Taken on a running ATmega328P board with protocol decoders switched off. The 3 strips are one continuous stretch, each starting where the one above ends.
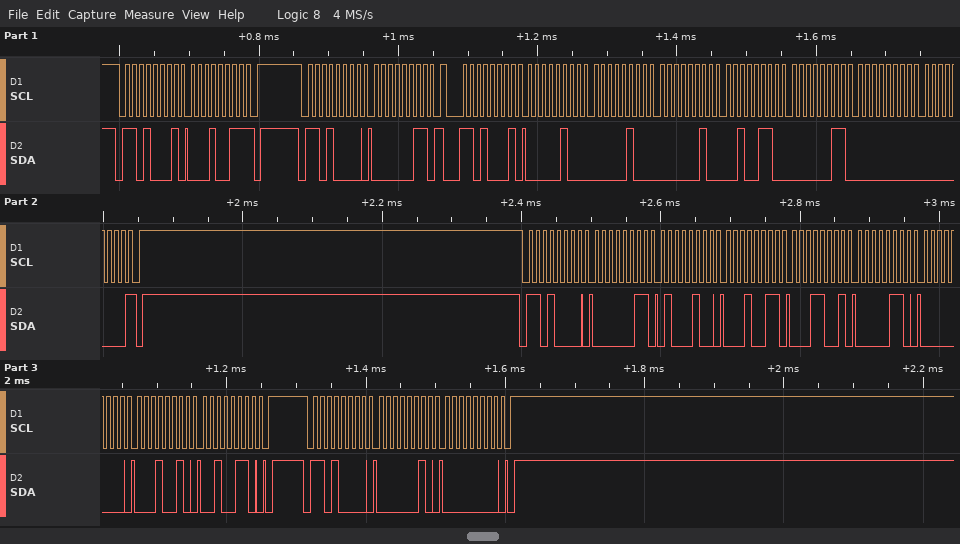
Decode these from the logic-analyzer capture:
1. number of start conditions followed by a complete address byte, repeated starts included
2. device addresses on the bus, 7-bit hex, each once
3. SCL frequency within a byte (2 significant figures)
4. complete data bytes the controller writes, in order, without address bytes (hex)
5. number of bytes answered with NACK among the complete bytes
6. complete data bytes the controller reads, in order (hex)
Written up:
5
0x68
100 kHz
03 03 44 13 19 06 00 12 26 02 00
2
13 04 04 02 26 03 00 00
